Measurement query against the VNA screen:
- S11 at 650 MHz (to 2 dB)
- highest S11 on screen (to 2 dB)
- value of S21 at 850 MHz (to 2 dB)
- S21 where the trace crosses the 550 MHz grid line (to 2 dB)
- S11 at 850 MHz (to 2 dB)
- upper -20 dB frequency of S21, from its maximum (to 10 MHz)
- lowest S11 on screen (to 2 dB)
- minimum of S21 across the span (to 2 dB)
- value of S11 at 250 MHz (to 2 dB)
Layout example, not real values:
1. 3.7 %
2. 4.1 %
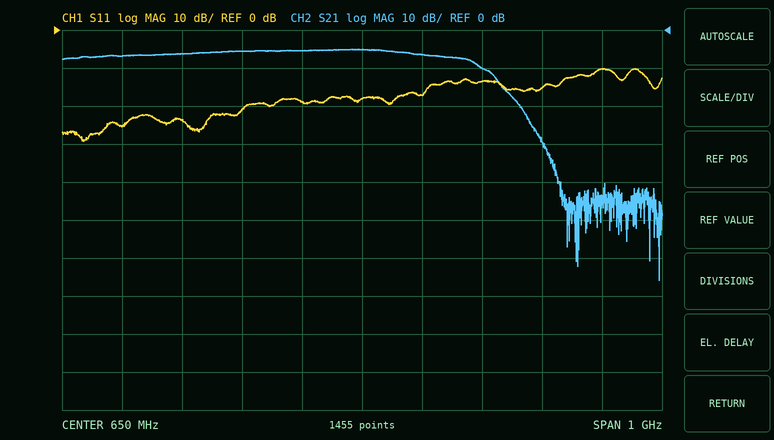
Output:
1. -18 dB
2. -10 dB
3. -10 dB
4. -6 dB
5. -14 dB
6. 930 MHz
7. -30 dB
8. -66 dB
9. -26 dB
